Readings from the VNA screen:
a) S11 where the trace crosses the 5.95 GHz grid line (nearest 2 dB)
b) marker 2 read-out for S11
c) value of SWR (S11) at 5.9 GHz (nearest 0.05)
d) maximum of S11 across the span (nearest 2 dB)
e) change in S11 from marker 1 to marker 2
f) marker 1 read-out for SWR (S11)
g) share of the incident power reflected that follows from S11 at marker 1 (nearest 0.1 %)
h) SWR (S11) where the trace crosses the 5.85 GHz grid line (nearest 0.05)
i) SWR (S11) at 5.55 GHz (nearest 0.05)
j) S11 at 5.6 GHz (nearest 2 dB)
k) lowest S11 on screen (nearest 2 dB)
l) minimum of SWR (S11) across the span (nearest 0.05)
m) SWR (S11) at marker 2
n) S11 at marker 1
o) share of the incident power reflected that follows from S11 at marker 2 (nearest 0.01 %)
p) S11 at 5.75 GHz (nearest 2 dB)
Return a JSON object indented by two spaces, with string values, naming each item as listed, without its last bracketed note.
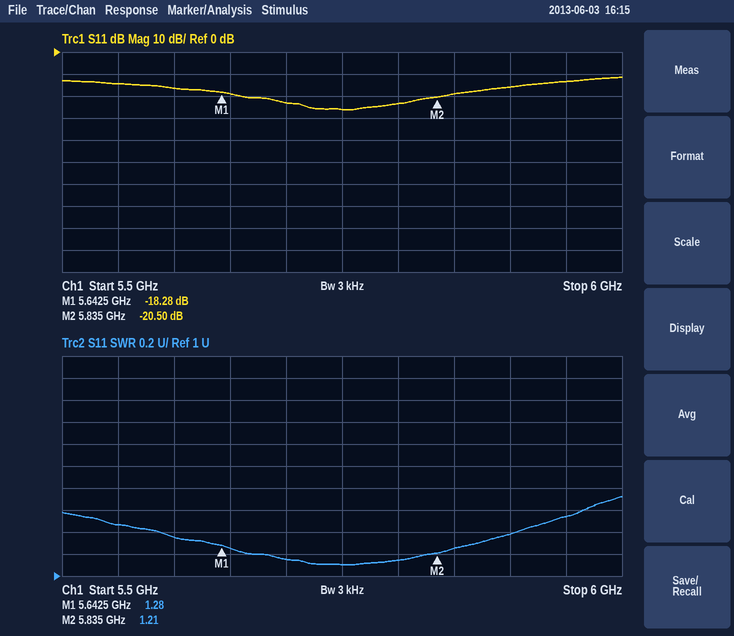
{
  "S11 where the trace crosses the 5.95 GHz grid line": "-14 dB",
  "marker 2 read-out for S11": "-20.50 dB",
  "value of SWR (S11) at 5.9 GHz": "1.40",
  "maximum of S11 across the span": "-12 dB",
  "change in S11 from marker 1 to marker 2": "-2.22 dB",
  "marker 1 read-out for SWR": "1.28",
  "share of the incident power reflected that follows from S11 at marker 1": "1.5 %",
  "SWR (S11) where the trace crosses the 5.85 GHz grid line": "1.25",
  "SWR (S11) at 5.55 GHz": "1.45",
  "S11 at 5.6 GHz": "-16 dB",
  "lowest S11 on screen": "-26 dB",
  "minimum of SWR (S11) across the span": "1.10",
  "SWR (S11) at marker 2": "1.21",
  "S11 at marker 1": "-18.28 dB",
  "share of the incident power reflected that follows from S11 at marker 2": "0.89 %",
  "S11 at 5.75 GHz": "-26 dB"
}
